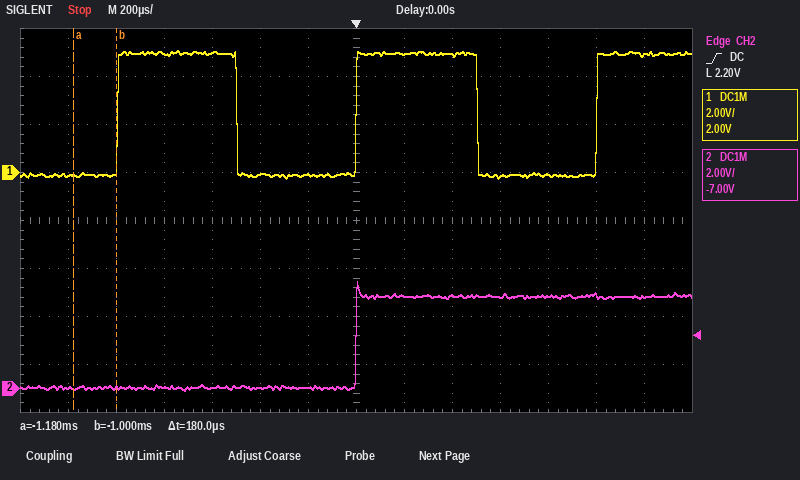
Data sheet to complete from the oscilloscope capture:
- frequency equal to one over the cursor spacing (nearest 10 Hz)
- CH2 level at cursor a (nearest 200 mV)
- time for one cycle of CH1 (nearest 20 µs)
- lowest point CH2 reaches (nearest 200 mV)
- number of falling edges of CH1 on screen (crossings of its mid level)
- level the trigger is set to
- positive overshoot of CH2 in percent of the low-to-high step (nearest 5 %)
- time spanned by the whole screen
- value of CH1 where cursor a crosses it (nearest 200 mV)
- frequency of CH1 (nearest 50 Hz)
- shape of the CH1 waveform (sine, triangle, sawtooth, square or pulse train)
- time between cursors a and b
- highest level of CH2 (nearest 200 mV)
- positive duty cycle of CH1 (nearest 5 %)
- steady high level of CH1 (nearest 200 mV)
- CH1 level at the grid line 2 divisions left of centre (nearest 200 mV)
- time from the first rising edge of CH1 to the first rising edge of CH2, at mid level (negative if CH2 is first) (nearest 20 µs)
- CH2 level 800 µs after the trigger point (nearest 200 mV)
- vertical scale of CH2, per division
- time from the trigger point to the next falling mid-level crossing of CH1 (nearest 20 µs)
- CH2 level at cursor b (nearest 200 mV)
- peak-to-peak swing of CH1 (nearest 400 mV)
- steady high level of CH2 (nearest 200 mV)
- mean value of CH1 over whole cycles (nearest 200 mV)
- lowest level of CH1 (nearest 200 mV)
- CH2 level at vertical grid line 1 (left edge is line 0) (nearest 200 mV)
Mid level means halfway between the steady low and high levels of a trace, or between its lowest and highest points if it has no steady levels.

5.56 kHz
0.0 V
1.00 ms
0.0 V
2
2.20 V
15 %
2.8 ms
-200 mV
1.00 kHz
square
180 µs
4.4 V
50 %
5.0 V
0.0 V
+1.00 ms
3.8 V
2 V
500 µs
0.0 V
5.2 V
3.8 V
2.4 V
-200 mV
0.0 V
